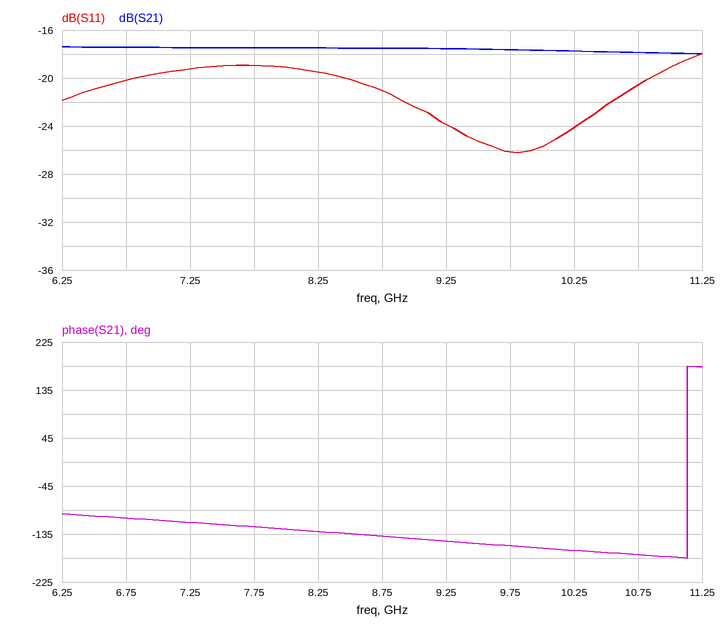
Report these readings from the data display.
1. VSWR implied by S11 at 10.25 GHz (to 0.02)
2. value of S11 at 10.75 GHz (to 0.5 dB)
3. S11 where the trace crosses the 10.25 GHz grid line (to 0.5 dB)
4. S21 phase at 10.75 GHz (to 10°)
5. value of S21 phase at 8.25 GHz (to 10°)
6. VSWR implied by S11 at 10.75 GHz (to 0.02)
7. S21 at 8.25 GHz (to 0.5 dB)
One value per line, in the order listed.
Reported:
1.14
-20.5 dB
-24.0 dB
-170°
-130°
1.20
-17.5 dB
